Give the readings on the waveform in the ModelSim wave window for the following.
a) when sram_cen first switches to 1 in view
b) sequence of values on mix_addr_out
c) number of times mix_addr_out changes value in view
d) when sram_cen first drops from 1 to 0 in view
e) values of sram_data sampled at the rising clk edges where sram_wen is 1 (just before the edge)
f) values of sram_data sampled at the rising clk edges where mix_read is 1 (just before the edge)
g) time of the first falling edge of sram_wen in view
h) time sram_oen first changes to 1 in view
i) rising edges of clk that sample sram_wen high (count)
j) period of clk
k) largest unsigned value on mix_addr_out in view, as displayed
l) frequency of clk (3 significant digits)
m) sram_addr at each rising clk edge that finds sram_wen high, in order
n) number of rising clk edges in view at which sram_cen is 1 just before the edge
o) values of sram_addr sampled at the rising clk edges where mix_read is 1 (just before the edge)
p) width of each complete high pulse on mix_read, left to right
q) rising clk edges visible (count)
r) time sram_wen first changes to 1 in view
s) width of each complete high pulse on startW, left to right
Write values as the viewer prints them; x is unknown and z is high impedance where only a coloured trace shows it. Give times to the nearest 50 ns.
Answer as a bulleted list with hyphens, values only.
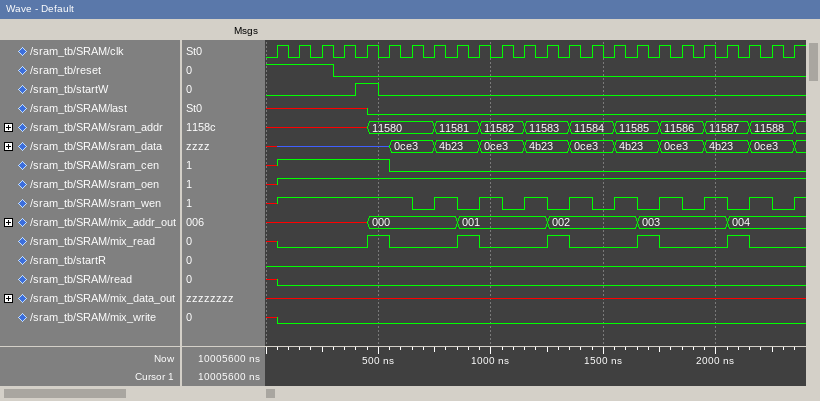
- 50 ns
- x, 000, 001, 002, 003, 004
- 5
- 550 ns
- z, z, z, z, z, 0ce3, 4b23, 0ce3, 4b23, 0ce3, 4b23, 0ce3, 4b23, 0ce3
- z, 4b23, 4b23, 4b23, 4b23
- 650 ns
- 50 ns
- 14
- 100 ns
- 004
- 10.0 MHz
- x, x, x, x, 11580, 11580, 11581, 11582, 11583, 11584, 11585, 11586, 11587, 11588
- 5
- 11580, 11581, 11583, 11585, 11587
- 100 ns, 100 ns, 100 ns, 100 ns, 100 ns
- 24
- 50 ns
- 100 ns
